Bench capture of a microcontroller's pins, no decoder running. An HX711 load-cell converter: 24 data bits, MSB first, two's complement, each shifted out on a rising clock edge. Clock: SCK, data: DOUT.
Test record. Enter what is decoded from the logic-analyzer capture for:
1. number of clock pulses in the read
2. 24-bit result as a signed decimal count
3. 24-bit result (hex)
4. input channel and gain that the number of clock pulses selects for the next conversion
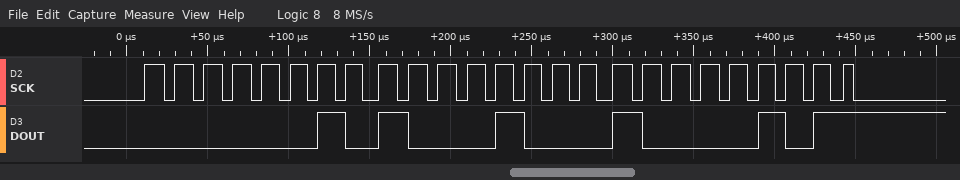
25
166021
0x028885
channel A, gain 128
